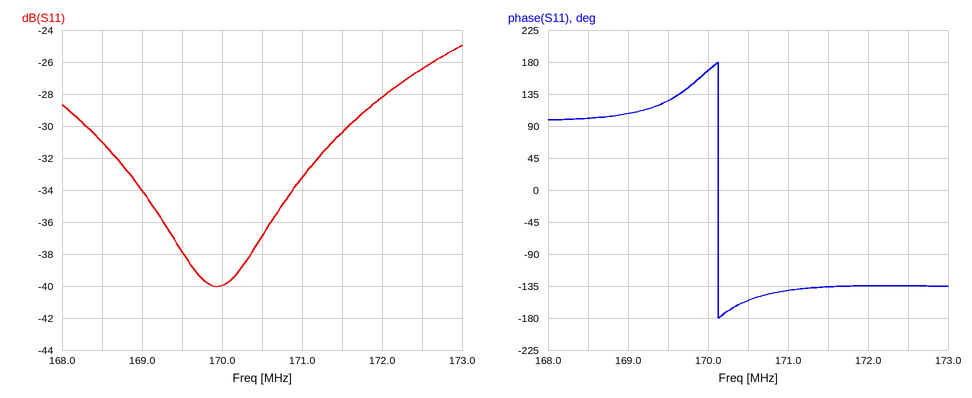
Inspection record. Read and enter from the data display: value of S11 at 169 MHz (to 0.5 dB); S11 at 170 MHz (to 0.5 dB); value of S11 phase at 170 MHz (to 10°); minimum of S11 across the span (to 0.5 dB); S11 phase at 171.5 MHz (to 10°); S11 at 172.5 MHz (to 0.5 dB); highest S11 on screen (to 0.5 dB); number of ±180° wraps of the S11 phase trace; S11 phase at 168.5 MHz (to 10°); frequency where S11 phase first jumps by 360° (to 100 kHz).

-34.0 dB
-40.0 dB
170°
-40.0 dB
-140°
-26.5 dB
-25.0 dB
1
100°
170.1 MHz
